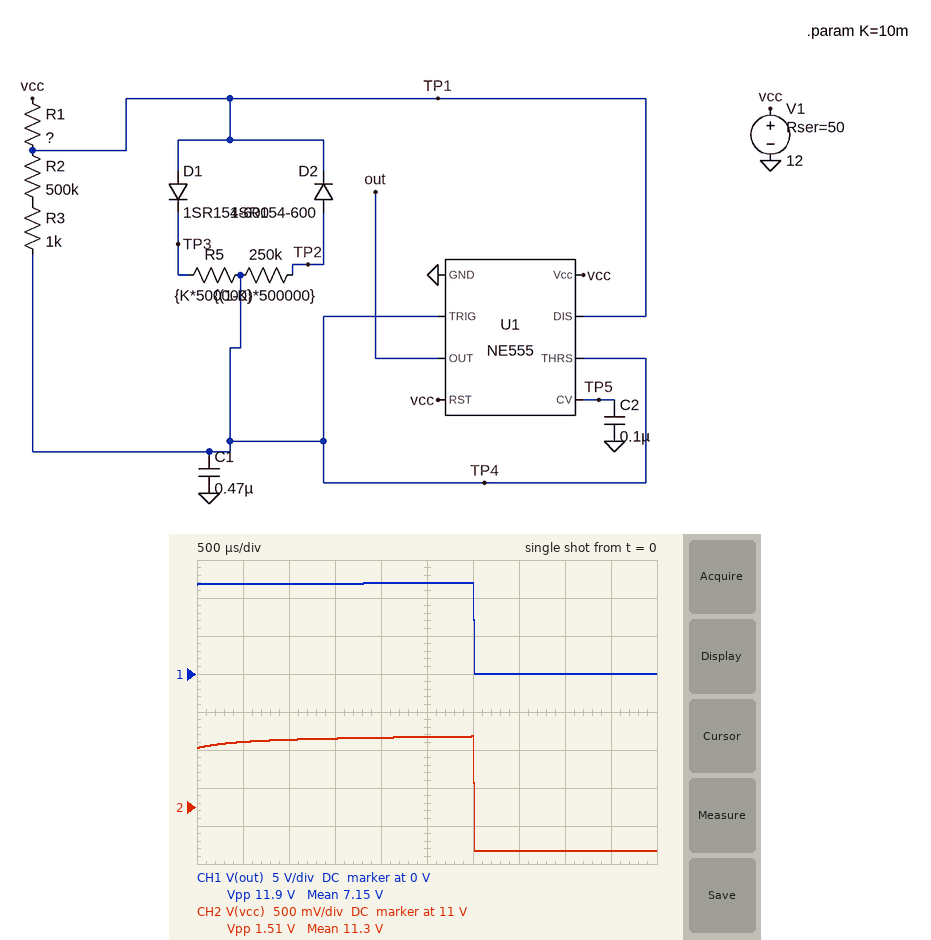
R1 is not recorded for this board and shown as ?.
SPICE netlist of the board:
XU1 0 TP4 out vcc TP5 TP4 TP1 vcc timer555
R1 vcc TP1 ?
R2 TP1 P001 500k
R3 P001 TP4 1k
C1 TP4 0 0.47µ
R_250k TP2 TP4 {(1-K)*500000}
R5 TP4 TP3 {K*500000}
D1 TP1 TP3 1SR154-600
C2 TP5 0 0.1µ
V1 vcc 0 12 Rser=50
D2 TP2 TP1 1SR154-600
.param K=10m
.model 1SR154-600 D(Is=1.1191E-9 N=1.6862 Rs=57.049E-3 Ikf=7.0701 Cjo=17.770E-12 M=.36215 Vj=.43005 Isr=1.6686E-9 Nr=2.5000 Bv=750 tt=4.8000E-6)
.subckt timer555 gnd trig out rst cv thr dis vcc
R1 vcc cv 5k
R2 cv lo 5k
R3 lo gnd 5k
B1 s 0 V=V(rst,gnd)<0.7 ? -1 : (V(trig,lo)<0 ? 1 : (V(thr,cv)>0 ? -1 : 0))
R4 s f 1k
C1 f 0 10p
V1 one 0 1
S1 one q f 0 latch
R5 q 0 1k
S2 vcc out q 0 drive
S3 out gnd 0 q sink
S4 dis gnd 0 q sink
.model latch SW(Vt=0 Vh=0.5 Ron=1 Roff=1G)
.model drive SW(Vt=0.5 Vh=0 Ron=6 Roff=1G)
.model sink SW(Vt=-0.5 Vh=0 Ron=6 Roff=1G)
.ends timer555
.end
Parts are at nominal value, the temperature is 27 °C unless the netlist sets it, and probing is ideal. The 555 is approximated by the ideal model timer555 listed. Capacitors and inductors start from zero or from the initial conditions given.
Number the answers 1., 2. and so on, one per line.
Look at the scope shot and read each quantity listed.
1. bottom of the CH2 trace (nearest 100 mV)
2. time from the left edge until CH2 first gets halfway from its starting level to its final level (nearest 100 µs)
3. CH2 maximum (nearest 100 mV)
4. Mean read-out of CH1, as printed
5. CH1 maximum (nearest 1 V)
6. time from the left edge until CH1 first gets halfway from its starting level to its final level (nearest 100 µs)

1. 10.4 V
2. 3.0 ms
3. 11.9 V
4. 7.15 V
5. 12 V
6. 3.0 ms
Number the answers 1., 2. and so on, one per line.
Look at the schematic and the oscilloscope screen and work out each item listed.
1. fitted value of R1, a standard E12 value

1. 330 Ω
